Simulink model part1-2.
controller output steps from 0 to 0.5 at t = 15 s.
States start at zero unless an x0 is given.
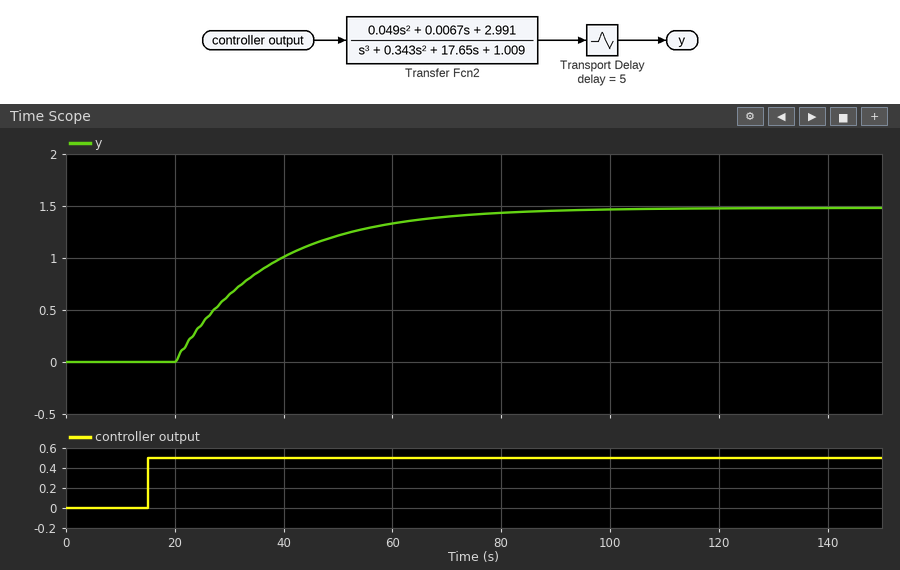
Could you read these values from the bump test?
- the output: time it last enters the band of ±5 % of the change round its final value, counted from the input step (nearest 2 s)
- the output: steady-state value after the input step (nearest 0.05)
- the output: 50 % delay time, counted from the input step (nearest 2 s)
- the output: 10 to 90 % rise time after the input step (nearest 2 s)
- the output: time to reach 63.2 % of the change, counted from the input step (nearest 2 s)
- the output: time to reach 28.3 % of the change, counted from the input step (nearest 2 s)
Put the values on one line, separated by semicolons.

58 s; 1.50; 18 s; 38 s; 22 s; 10 s
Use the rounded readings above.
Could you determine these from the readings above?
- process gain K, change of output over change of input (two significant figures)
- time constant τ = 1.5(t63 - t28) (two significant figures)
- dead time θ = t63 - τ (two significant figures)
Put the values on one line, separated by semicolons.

3.0; 18 s; 4.0 s
